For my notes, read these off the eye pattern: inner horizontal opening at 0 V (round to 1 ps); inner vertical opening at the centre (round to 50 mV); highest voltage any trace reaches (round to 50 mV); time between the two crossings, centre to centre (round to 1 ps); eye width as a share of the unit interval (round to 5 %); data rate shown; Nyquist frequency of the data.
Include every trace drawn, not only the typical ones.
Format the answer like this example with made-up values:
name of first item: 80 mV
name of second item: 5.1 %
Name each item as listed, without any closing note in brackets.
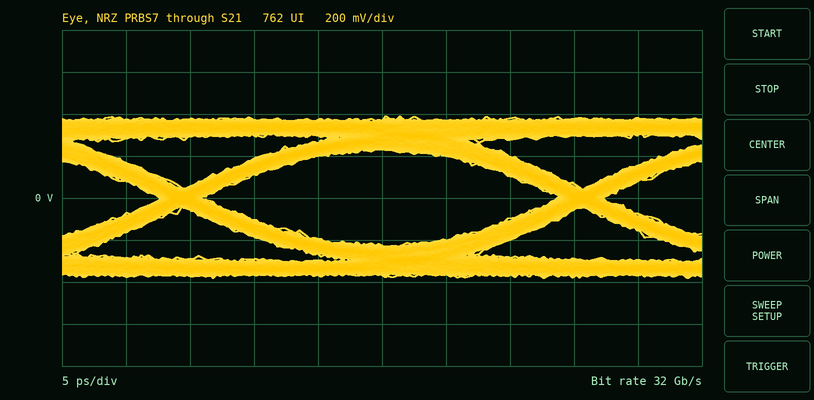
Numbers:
inner horizontal opening at 0 V: 28 ps
inner vertical opening at the centre: 450 mV
highest voltage any trace reaches: 400 mV
time between the two crossings, centre to centre: 31 ps
eye width as a share of the unit interval: 90 %
data rate shown: 32 Gb/s
Nyquist frequency of the data: 16 GHz
